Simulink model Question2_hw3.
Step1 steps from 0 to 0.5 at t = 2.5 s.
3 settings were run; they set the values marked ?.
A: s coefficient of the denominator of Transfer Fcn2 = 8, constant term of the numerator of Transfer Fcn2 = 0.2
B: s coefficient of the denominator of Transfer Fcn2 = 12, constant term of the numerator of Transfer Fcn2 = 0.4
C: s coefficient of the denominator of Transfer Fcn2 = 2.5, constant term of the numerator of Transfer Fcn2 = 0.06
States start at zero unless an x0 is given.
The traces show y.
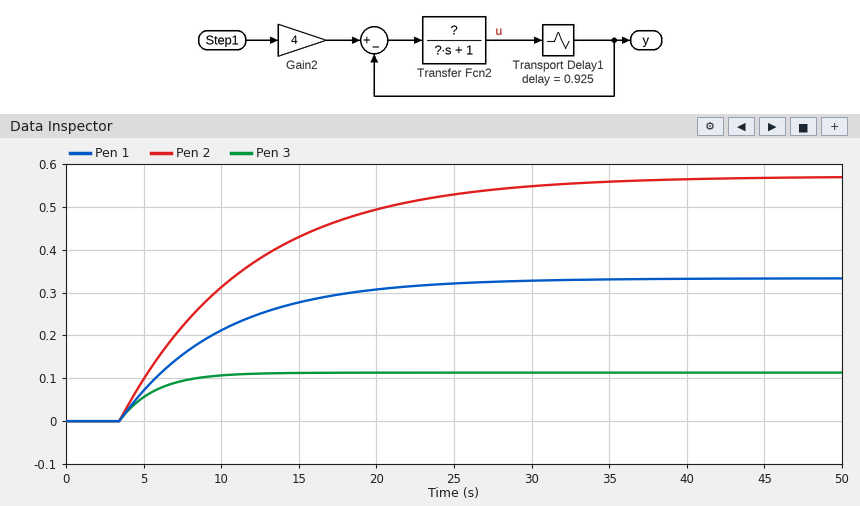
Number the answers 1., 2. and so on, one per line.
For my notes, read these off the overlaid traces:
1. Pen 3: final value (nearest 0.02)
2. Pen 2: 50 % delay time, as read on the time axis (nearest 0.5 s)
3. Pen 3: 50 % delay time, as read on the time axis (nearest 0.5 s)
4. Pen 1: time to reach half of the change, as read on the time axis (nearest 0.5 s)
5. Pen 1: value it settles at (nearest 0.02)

1. 0.12
2. 9.0 s
3. 5.0 s
4. 8.0 s
5. 0.34
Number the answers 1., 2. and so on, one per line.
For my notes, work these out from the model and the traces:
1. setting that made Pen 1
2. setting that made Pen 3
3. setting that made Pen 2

1. A
2. C
3. B
